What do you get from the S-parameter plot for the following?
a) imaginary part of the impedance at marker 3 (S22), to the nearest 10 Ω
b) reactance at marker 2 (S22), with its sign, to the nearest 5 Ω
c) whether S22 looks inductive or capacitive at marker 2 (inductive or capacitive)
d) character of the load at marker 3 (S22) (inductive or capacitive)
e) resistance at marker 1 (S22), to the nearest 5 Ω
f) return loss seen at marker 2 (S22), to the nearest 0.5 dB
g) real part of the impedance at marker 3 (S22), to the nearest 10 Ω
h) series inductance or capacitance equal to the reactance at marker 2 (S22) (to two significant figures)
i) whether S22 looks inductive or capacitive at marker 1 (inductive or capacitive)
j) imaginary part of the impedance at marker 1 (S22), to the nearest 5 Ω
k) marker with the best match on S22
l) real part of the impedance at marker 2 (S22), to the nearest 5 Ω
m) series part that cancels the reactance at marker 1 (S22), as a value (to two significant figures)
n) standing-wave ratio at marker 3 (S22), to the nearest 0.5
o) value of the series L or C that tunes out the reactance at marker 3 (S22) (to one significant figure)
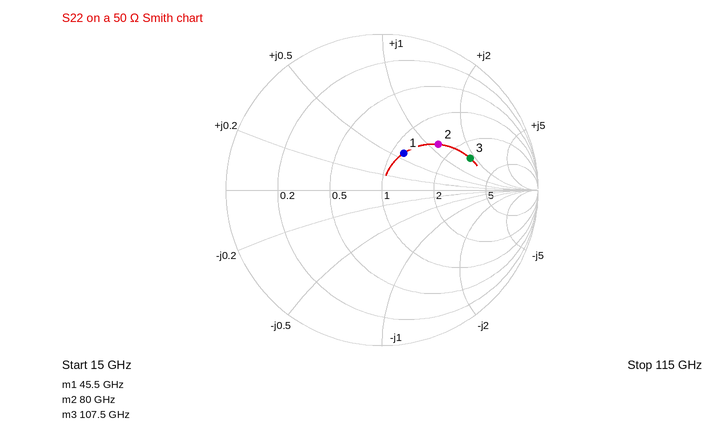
+90 Ω
+60 Ω
inductive
inductive
60 Ω
6.5 dB
140 Ω
120 pH
inductive
+30 Ω
marker 1
80 Ω
120 fF
4.0
20 fF
